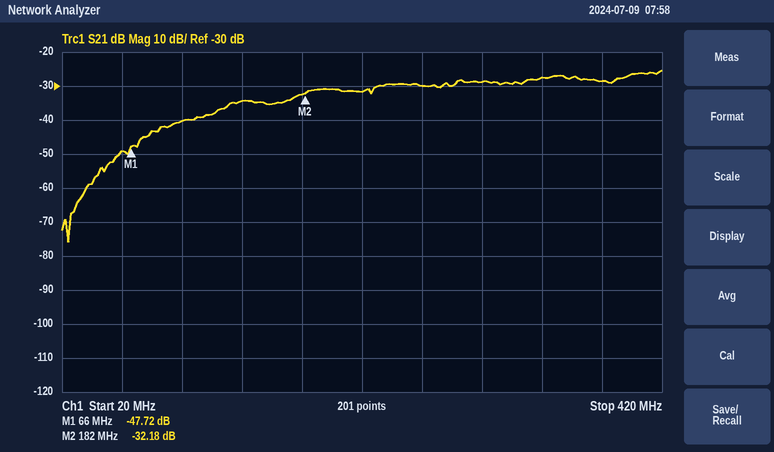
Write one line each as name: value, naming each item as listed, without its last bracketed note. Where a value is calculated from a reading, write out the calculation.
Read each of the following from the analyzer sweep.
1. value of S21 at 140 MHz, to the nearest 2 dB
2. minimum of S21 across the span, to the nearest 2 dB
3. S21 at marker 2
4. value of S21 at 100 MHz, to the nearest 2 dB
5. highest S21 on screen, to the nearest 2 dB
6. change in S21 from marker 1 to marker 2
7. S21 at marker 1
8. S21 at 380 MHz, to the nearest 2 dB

value of S21 at 140 MHz, to the nearest 2 dB: -34 dB
minimum of S21 across the span, to the nearest 2 dB: -76 dB
S21 at marker 2: -32.18 dB
value of S21 at 100 MHz, to the nearest 2 dB: -40 dB
highest S21 on screen, to the nearest 2 dB: -26 dB
change in S21 from marker 1 to marker 2: -32.18 − (-47.72) = 15.54 dB
S21 at marker 1: -47.72 dB
S21 at 380 MHz, to the nearest 2 dB: -28 dB
